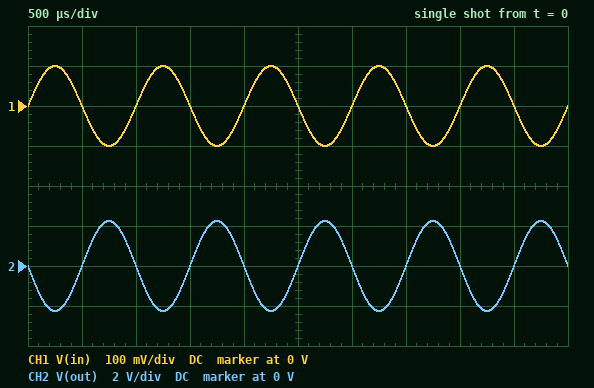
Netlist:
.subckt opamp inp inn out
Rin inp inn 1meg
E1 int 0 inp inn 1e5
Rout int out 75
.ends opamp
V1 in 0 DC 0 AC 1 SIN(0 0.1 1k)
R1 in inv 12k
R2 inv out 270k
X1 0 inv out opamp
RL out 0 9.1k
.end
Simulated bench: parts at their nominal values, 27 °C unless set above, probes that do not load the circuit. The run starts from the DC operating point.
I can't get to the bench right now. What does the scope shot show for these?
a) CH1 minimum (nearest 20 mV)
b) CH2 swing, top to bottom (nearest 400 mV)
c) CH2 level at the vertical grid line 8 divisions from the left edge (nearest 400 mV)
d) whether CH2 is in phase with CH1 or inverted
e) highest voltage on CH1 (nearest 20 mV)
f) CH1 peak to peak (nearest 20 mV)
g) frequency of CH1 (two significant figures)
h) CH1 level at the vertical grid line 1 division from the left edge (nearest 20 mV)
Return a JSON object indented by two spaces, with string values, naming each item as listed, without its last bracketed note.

{
  "CH1 minimum": "-100 mV",
  "CH2 swing, top to bottom": "4.4 V",
  "CH2 level at the vertical grid line 8 divisions from the left edge": "0 V",
  "whether CH2 is in phase with CH1 or inverted": "inverted",
  "highest voltage on CH1": "100 mV",
  "CH1 peak to peak": "200 mV",
  "frequency of CH1": "1.0 kHz",
  "CH1 level at the vertical grid line 1 division from the left edge": "0 V"
}
